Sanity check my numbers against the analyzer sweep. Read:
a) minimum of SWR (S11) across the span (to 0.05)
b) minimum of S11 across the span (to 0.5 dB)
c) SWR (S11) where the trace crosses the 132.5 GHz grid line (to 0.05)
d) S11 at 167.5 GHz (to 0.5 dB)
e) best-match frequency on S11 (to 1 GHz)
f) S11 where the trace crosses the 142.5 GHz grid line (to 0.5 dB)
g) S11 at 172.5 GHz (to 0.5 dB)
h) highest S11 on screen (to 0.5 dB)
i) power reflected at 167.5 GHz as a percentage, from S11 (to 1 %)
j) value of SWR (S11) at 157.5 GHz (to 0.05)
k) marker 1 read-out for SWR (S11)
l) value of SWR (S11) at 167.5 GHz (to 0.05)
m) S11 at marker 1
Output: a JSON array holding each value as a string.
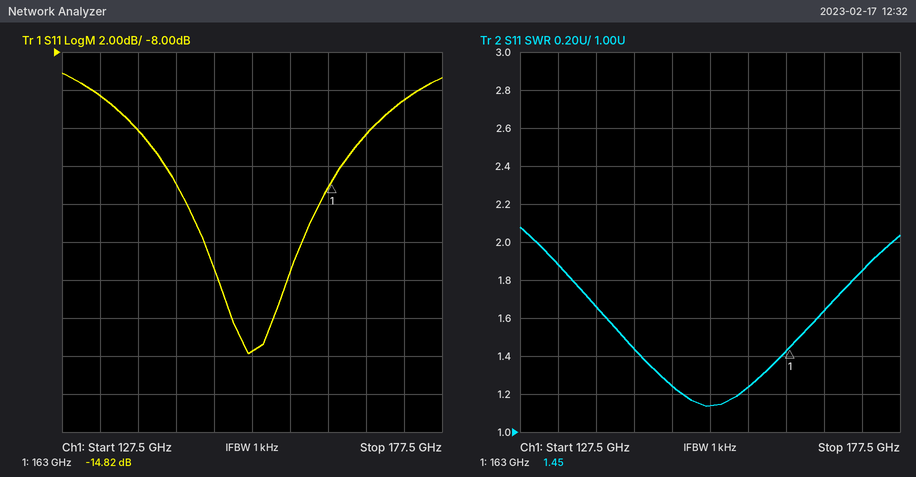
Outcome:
["1.15", "-24.0 dB", "1.90", "-12.5 dB", "152 GHz", "-15.0 dB", "-10.5 dB", "-9.0 dB", "6 %", "1.25", "1.45", "1.65", "-14.82 dB"]
